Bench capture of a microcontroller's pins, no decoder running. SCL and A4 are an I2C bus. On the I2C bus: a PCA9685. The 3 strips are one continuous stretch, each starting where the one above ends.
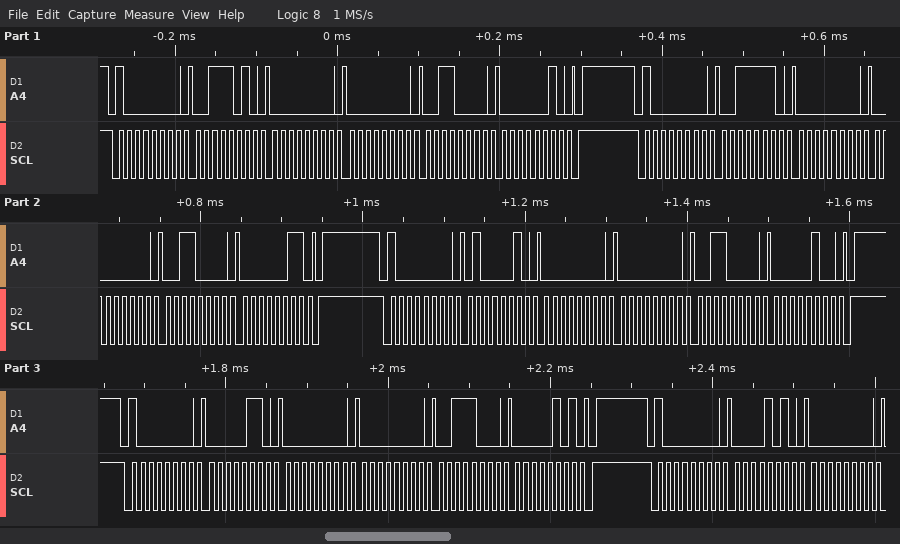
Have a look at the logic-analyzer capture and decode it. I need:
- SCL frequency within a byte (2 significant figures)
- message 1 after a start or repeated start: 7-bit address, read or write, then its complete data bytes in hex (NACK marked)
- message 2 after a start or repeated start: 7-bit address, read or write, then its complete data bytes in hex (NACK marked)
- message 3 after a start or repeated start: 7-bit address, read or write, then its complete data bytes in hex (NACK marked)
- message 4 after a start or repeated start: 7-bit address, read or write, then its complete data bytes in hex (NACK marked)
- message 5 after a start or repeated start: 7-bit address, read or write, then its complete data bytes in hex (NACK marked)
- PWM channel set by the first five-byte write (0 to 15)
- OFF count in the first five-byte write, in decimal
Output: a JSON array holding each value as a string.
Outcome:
["100 kHz", "0x40 write: 3A 00 00 30 02", "0x40 write: 3E 00 00 30 03", "0x40 write: 42 00 00 30 04", "0x40 write: 06 00 00 38 05", "0x40 write: 0A 00", "13", "560"]
